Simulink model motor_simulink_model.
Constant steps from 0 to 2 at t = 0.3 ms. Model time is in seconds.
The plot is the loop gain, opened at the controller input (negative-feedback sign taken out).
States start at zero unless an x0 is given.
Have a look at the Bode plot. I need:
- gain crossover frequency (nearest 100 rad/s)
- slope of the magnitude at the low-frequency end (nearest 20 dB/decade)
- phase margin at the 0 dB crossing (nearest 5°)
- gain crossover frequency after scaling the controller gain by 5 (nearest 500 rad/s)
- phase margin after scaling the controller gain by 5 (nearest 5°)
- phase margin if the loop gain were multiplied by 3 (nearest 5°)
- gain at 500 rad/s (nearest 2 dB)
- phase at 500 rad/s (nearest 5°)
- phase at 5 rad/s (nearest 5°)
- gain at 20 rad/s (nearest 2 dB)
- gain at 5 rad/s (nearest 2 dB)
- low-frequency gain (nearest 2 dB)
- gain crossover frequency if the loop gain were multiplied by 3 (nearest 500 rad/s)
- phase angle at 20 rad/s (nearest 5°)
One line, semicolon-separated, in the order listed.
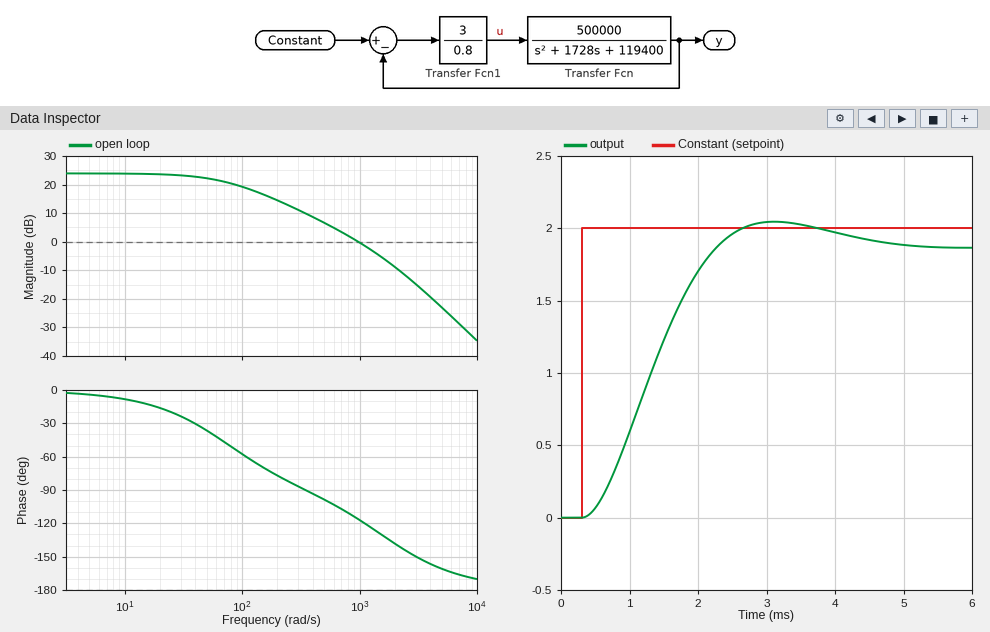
1000 rad/s; 0 dB/decade; 65°; 3000 rad/s; 30°; 40°; 6 dB; -100°; -5°; 24 dB; 24 dB; 24 dB; 2000 rad/s; -15°
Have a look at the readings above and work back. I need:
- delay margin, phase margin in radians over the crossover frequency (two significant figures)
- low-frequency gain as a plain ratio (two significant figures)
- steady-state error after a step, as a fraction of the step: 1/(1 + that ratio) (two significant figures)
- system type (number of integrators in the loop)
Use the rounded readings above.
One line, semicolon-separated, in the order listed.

0.0011 s; 16; 0.059; 0
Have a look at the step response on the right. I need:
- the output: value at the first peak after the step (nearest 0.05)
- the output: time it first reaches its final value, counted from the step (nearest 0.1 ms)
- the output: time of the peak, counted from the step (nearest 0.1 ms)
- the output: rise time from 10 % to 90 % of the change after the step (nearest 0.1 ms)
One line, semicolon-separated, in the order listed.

2.05; 2.0 ms; 2.8 ms; 1.3 ms
